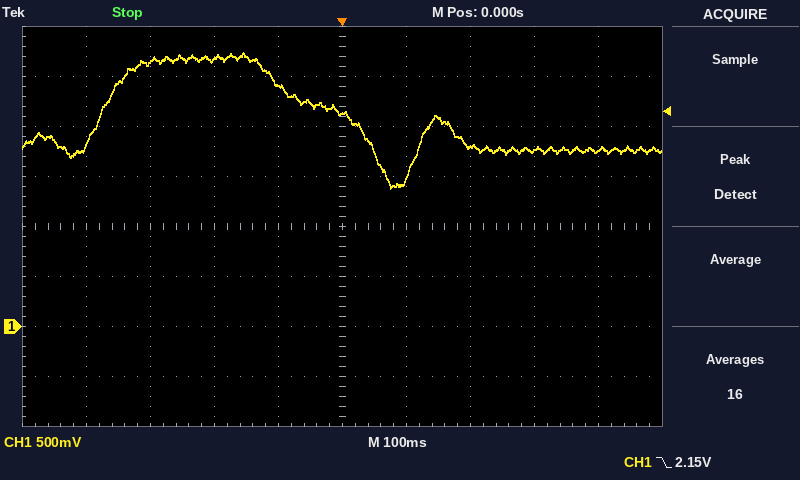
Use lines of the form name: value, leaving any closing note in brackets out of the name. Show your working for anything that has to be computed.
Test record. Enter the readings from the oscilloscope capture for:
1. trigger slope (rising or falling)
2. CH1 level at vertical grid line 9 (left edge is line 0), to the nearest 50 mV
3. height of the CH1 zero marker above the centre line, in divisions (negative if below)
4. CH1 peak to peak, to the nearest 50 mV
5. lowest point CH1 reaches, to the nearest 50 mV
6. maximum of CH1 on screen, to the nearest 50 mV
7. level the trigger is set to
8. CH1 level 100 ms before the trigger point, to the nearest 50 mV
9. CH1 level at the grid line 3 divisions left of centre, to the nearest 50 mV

trigger slope: falling
CH1 level at vertical grid line 9 (left edge is line 0), to the nearest 50 mV: 1.75 V
height of the CH1 zero marker above the centre line, in divisions: -2.0 div
CH1 peak to peak, to the nearest 50 mV: 2.75 V − (1.40 V) = 1.35 V
lowest point CH1 reaches, to the nearest 50 mV: 1.40 V
maximum of CH1 on screen, to the nearest 50 mV: 2.75 V
level the trigger is set to: 2.15 V
CH1 level 100 ms before the trigger point, to the nearest 50 mV: 2.40 V
CH1 level at the grid line 3 divisions left of centre, to the nearest 50 mV: 2.65 V
